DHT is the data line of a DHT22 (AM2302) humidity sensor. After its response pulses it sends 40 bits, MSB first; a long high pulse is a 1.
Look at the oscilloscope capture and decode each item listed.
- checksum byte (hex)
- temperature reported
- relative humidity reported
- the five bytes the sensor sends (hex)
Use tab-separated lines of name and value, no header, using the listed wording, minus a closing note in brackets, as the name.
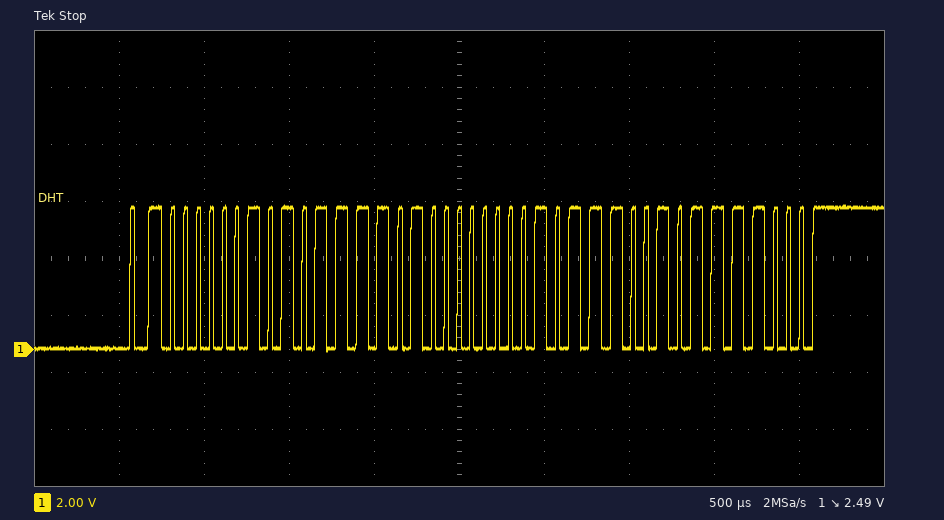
checksum byte	0x78
temperature reported	18.5 °C
relative humidity reported	70.1 %
the five bytes the sensor sends	02 BD 00 B9 78
